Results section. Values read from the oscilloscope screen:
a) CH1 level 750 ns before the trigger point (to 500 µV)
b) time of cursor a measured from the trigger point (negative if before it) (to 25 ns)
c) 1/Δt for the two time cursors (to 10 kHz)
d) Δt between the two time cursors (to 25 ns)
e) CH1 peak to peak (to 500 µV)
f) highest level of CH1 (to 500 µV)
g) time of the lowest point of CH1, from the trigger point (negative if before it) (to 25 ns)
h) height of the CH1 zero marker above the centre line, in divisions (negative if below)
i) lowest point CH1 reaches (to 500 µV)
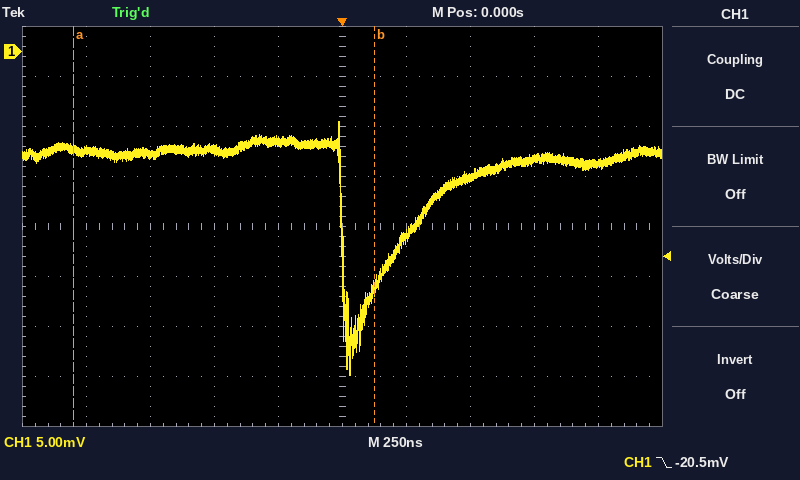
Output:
-10.5 mV
-1.050 µs
850 kHz
1.175 µs
25.5 mV
-7.0 mV
+25 ns
+3.5 div
-32.5 mV
